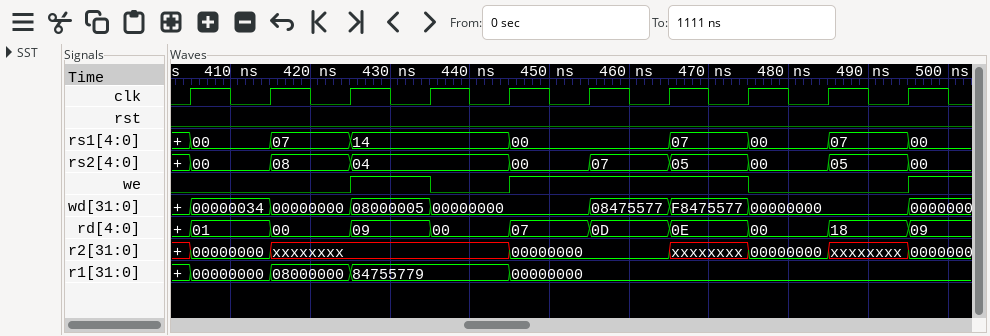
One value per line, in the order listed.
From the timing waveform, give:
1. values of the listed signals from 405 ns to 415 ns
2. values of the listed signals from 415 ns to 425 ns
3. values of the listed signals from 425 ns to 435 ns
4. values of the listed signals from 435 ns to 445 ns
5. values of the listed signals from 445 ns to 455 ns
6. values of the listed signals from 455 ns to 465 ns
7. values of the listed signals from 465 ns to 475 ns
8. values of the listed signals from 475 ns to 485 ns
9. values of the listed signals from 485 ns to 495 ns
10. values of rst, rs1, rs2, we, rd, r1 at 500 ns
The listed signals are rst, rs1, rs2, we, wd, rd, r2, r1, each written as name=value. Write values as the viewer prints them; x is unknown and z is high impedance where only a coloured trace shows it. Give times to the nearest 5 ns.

rst=0, rs1=00, rs2=00, we=0, wd=00000034, rd=01, r2=00000000, r1=00000000
rst=0, rs1=07, rs2=08, we=0, wd=00000000, rd=00, r2=xxxxxxxx, r1=08000000
rst=0, rs1=14, rs2=04, we=1, wd=08000005, rd=09, r2=xxxxxxxx, r1=84755779
rst=0, rs1=14, rs2=04, we=0, wd=00000000, rd=00, r2=xxxxxxxx, r1=84755779
rst=0, rs1=00, rs2=00, we=1, wd=00000000, rd=07, r2=00000000, r1=00000000
rst=0, rs1=00, rs2=07, we=1, wd=08475577, rd=0D, r2=00000000, r1=00000000
rst=0, rs1=07, rs2=05, we=1, wd=F8475577, rd=0E, r2=xxxxxxxx, r1=00000000
rst=0, rs1=00, rs2=00, we=0, wd=00000000, rd=00, r2=00000000, r1=00000000
rst=0, rs1=07, rs2=05, we=0, wd=00000000, rd=18, r2=xxxxxxxx, r1=00000000
rst=0, rs1=00, rs2=00, we=1, rd=09, r1=00000000
